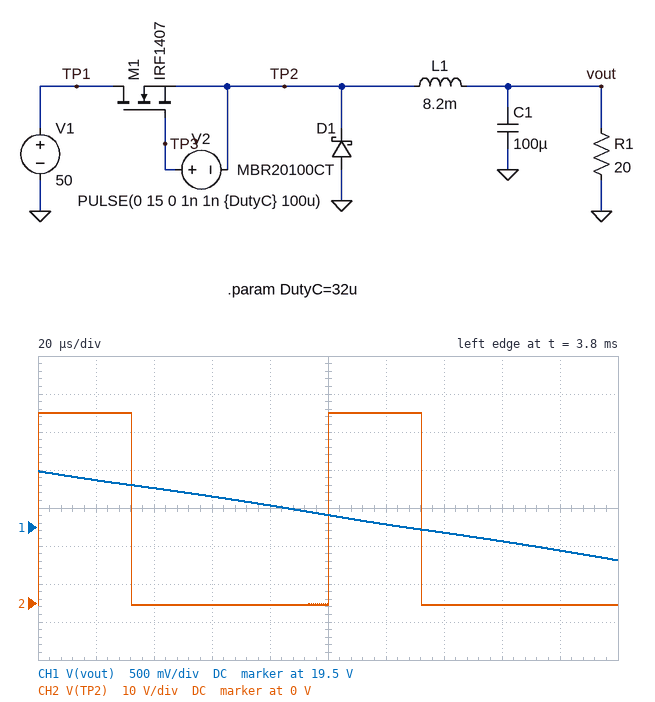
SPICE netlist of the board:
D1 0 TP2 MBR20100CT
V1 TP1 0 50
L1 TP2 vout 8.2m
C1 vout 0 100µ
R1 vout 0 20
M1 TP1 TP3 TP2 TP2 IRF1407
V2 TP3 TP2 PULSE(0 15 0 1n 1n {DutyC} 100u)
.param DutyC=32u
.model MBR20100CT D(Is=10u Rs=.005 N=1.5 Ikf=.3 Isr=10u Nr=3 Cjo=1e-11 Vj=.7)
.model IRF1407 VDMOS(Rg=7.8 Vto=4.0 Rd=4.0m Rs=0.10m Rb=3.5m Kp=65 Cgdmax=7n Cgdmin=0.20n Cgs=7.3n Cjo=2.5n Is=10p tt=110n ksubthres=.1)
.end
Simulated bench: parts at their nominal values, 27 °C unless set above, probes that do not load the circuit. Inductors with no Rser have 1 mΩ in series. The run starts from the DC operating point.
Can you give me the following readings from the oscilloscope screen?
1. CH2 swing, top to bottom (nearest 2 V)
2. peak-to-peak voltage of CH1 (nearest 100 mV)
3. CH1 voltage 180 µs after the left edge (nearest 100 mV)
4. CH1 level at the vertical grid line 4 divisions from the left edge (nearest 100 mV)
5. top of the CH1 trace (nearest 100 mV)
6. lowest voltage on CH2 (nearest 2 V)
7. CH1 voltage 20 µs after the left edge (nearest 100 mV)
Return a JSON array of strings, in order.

["50 V", "1.2 V", "19.2 V", "19.8 V", "20.2 V", "0 V", "20.1 V"]
